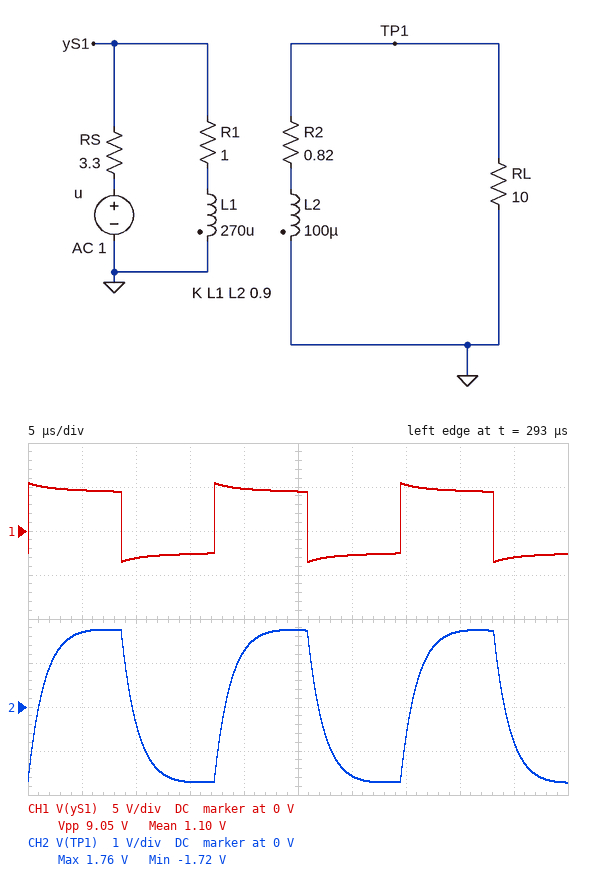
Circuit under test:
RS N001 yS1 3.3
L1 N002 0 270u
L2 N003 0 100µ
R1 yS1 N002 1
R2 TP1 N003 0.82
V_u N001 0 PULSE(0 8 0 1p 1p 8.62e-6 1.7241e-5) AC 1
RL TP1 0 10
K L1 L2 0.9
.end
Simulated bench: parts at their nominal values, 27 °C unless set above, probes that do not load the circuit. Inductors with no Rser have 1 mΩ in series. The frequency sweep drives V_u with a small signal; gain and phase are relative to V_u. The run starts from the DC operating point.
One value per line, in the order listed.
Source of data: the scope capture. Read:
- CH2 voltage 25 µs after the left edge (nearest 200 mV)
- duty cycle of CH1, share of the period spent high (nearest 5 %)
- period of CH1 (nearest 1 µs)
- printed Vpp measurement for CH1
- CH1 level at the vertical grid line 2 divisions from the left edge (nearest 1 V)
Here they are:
1.8 V
50 %
17 µs
9.05 V
-3 V
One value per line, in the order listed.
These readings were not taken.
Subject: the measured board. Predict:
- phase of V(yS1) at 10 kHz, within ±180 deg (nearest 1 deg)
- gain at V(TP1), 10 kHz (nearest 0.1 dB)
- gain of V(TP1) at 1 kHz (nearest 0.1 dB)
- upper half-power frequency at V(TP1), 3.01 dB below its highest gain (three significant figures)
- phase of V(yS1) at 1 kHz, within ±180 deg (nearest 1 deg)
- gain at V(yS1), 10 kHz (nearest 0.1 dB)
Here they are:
10 deg
-7.2 dB
-14.8 dB
106 kHz
36 deg
-1.0 dB
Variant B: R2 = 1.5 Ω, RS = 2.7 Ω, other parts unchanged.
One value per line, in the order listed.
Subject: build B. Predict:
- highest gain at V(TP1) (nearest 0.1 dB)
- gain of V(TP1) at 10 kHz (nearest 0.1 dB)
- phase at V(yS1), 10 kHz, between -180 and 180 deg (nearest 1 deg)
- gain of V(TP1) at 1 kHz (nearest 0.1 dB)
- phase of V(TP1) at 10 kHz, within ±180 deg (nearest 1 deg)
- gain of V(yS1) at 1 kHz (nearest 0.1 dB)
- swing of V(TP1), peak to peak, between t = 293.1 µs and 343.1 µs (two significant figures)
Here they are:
-7.4 dB
-7.5 dB
8 deg
-14.2 dB
6 deg
-6.3 dB
3.4 V
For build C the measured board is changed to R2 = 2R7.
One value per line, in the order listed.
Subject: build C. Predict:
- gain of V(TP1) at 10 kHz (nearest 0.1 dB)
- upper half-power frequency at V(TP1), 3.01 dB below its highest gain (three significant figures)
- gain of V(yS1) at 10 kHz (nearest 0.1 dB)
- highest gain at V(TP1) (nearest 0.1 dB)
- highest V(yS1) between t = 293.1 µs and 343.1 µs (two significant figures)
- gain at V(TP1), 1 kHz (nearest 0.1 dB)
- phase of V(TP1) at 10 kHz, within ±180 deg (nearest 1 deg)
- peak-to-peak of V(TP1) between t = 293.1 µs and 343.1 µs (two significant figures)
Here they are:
-8.4 dB
122 kHz
-0.9 dB
-8.3 dB
5.4 V
-16.1 dB
8 deg
3.0 V
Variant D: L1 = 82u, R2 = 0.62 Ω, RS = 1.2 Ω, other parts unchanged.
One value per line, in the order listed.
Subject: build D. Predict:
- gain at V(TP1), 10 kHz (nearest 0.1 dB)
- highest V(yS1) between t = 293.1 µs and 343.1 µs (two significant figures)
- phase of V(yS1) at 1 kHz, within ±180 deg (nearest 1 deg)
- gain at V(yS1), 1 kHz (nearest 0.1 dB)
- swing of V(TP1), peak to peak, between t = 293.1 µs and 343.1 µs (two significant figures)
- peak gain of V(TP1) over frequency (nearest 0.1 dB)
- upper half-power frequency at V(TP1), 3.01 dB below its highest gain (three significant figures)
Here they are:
-2.8 dB
6.4 V
14 deg
-6.0 dB
5.9 V
-2.5 dB
115 kHz
